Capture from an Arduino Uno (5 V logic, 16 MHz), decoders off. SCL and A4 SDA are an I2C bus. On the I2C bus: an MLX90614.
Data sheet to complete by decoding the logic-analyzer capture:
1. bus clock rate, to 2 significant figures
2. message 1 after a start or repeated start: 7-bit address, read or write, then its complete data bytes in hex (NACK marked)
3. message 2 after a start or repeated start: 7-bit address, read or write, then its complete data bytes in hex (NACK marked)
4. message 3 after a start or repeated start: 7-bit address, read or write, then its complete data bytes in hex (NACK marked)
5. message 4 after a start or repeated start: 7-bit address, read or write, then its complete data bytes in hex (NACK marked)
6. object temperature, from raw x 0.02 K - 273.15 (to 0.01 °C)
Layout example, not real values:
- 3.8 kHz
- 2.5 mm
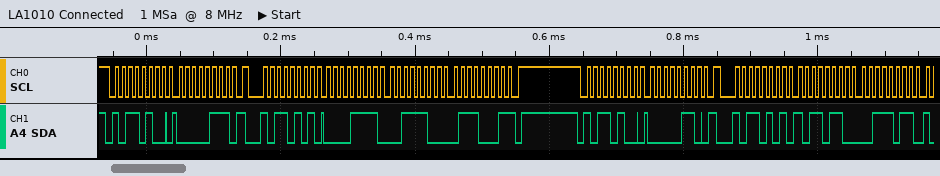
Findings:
- 100 kHz
- 0x5A write: 07
- 0x5A read: 0F 3C 71 NACK
- 0x5A write: 06
- 0x5A read: B6 3B
- 34.35 °C
